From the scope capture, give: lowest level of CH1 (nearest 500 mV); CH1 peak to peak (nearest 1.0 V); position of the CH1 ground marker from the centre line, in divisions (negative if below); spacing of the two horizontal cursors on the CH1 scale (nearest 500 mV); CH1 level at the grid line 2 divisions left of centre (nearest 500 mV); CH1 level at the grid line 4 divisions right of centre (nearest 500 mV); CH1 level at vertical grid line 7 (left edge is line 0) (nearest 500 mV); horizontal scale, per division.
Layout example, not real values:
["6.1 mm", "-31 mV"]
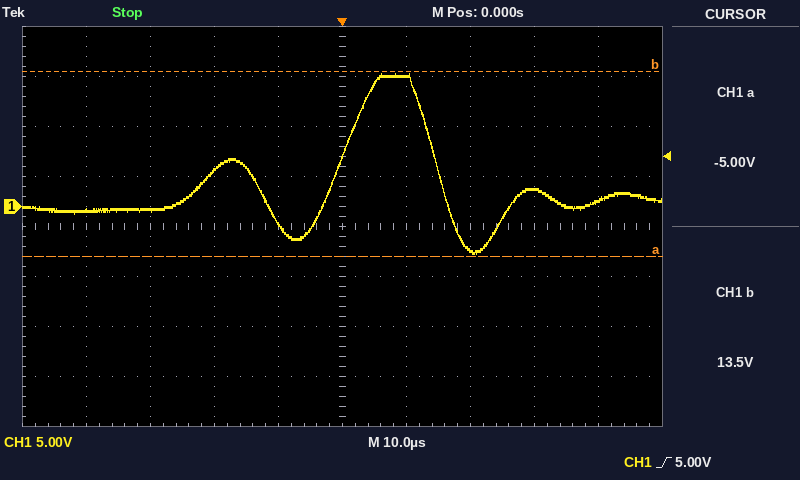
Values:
["-5.0 V", "18.0 V", "+0.4 div", "18.5 V", "3.5 V", "500 mV", "-4.5 V", "10 µs"]
